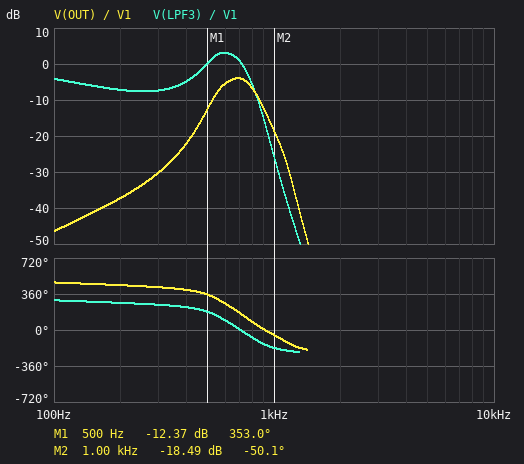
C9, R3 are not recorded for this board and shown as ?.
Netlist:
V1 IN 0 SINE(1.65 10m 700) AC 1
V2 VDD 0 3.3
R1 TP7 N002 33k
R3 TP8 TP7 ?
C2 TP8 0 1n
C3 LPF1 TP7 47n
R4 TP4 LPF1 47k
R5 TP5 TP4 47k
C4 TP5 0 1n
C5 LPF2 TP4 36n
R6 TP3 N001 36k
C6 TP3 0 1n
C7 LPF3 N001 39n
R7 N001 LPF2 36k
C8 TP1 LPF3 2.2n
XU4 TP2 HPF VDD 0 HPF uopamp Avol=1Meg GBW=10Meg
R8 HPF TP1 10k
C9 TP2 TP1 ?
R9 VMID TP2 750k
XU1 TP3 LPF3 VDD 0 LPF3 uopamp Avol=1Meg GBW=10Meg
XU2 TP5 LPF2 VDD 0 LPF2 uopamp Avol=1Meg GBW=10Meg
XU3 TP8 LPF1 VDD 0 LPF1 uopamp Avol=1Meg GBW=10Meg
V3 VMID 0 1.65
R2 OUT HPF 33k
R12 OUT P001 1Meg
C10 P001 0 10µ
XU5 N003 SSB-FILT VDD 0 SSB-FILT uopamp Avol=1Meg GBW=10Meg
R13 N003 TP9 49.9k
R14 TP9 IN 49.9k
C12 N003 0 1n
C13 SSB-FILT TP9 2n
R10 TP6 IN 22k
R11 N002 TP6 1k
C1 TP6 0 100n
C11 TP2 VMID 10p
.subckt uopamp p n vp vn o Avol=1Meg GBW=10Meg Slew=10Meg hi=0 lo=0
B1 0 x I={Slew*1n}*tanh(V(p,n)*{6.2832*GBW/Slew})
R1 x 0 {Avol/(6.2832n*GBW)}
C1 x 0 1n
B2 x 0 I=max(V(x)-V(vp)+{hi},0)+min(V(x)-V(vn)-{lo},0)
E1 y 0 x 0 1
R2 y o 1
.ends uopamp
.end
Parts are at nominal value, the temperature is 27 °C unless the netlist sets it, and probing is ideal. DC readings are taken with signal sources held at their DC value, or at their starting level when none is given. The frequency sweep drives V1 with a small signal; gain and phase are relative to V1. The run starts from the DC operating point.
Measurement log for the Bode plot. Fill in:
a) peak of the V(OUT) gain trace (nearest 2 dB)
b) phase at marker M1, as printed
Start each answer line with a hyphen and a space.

- -4 dB
- 353.0 deg
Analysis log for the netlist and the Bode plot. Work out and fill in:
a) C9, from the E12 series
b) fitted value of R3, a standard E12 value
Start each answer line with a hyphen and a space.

- 1.2 nF
- 22 kΩ
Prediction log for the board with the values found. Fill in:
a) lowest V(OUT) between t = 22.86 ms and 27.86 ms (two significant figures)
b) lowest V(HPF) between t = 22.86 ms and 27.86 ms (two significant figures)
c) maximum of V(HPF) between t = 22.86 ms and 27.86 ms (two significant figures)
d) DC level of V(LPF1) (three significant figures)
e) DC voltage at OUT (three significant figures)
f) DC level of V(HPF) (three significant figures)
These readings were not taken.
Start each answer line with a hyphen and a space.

- 1.6 V
- 1.6 V
- 1.7 V
- 1.65 V
- 1.65 V
- 1.65 V
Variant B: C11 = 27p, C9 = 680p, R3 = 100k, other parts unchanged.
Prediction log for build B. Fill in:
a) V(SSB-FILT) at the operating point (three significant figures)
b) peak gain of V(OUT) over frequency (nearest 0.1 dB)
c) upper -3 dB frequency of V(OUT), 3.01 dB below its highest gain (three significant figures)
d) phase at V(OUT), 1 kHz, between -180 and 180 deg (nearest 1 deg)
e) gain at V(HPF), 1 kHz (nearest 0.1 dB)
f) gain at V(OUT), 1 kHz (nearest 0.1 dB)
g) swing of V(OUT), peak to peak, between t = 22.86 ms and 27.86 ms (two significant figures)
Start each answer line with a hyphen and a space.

- 1.65 V
- -18.9 dB
- 647 Hz
- -64 deg
- -48.1 dB
- -48.4 dB
- 1.1 mV
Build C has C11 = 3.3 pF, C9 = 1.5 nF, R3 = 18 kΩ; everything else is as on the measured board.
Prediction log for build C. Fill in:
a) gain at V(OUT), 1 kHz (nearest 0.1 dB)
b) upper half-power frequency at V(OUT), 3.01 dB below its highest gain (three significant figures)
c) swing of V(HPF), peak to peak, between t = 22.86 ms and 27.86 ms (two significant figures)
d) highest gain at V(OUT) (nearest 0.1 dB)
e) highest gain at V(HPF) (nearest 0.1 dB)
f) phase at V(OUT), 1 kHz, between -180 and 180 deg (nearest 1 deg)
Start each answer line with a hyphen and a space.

- -11.0 dB
- 845 Hz
- 16 mV
- -2.2 dB
- -1.9 dB
- -61 deg
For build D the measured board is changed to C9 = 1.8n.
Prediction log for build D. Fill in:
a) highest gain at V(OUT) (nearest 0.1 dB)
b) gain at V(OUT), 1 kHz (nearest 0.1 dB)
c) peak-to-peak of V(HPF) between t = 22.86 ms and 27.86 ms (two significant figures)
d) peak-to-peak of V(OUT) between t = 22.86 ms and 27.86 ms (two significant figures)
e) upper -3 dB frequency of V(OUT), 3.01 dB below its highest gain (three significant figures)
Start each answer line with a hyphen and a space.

- 2.3 dB
- -15.4 dB
- 27 mV
- 26 mV
- 834 Hz
